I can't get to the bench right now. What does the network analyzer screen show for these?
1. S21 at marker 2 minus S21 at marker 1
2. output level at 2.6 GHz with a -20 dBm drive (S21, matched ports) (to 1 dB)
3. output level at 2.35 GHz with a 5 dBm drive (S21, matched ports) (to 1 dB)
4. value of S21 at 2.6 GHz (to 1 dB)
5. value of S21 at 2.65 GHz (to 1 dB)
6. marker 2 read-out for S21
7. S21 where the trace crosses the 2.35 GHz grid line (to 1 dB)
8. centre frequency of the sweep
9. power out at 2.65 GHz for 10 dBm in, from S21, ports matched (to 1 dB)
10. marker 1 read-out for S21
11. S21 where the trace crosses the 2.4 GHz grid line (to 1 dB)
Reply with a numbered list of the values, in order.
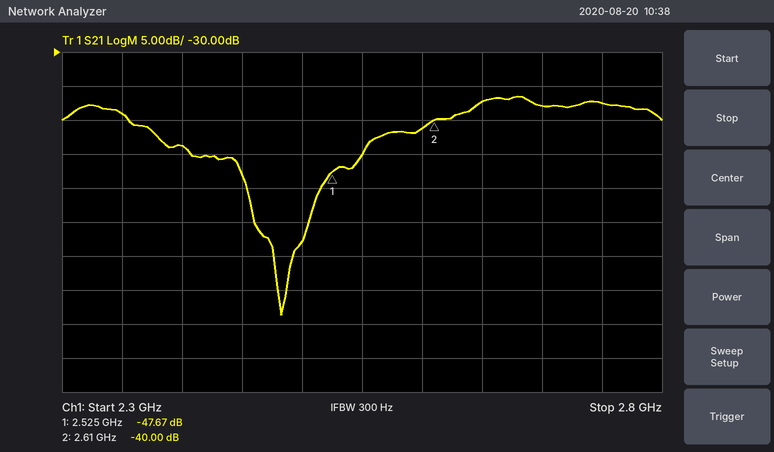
1. 7.67 dB
2. -61 dBm
3. -34 dBm
4. -41 dB
5. -37 dB
6. -40.00 dB
7. -39 dB
8. 2.55 GHz
9. -27 dBm
10. -47.67 dB
11. -44 dB
